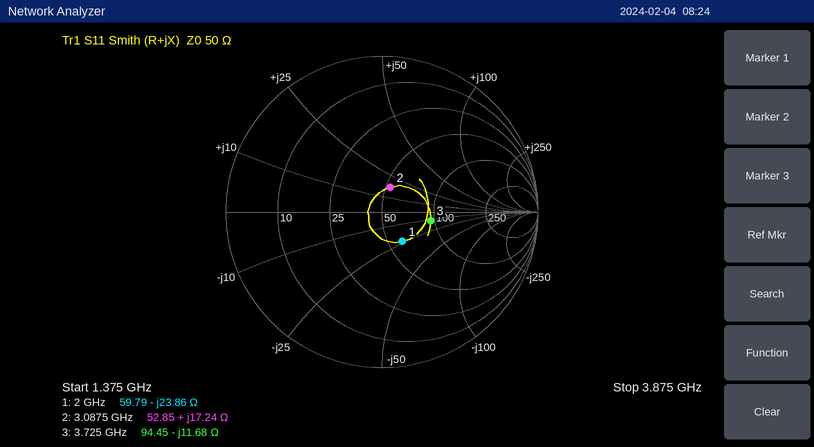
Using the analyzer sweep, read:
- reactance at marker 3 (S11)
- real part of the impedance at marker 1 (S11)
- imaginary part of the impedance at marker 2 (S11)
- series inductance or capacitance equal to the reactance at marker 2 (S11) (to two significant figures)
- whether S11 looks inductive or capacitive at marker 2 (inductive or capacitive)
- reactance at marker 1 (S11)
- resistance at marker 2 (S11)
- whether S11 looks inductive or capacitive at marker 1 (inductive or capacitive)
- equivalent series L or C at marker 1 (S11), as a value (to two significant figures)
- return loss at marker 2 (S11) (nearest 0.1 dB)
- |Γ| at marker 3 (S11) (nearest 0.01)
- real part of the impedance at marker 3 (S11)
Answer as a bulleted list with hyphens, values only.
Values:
- -11.68 Ω
- 59.79 Ω
- +17.24 Ω
- 890 pH
- inductive
- -23.86 Ω
- 52.85 Ω
- capacitive
- 3.3 pF
- 15.5 dB
- 0.32
- 94.45 Ω
